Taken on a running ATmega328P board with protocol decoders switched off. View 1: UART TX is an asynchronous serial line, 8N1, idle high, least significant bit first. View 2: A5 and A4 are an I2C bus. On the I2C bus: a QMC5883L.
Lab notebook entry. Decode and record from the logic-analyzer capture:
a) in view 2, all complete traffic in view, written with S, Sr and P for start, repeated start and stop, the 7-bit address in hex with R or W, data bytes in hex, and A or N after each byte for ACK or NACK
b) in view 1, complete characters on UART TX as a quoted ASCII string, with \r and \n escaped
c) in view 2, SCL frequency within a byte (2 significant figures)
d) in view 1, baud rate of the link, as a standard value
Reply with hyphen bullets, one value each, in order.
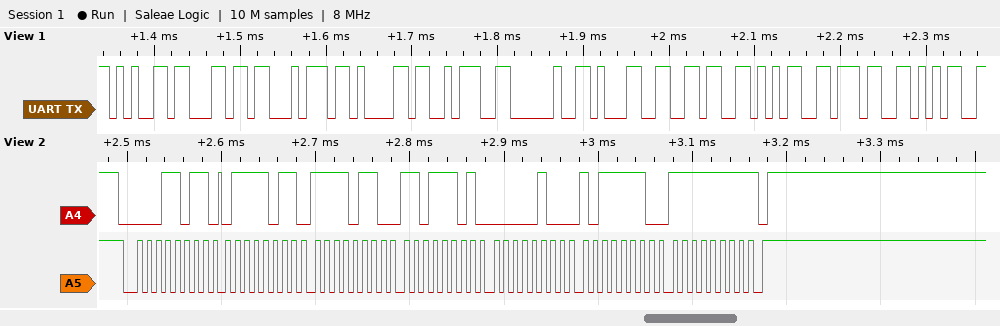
- S 0DR A 7B A F6 A DD A 04 A BE A FF N P
- "elta: 16575"
- 100 kHz
- 115200 baud
